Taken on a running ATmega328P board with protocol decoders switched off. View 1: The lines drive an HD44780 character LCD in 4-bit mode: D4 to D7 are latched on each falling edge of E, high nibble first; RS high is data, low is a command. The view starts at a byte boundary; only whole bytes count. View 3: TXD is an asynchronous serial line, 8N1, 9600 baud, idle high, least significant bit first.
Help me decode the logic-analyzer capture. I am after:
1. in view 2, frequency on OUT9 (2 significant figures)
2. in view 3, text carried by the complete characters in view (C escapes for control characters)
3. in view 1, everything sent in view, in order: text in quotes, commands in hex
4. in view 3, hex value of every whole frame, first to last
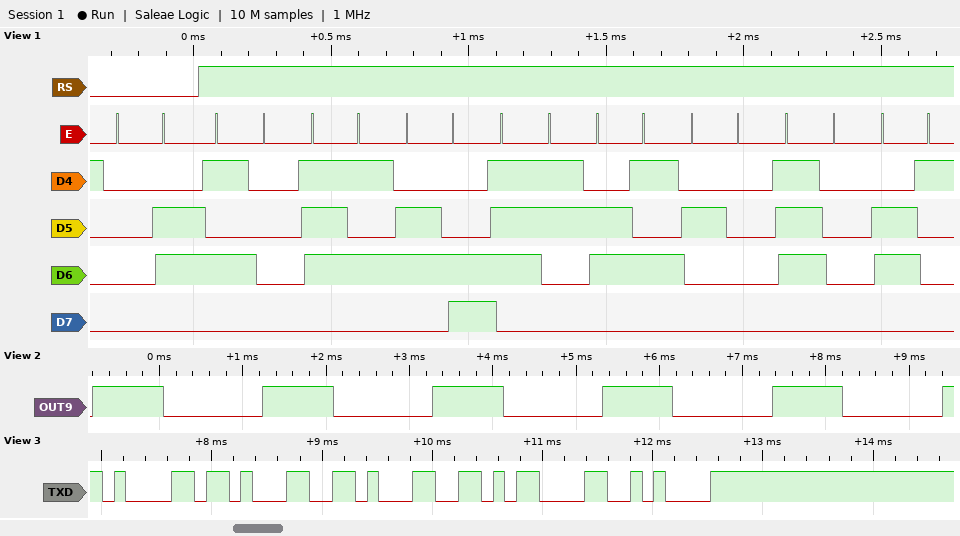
490 Hz
"a11\r\n"
0x06 "Pulse pa"
61 31 31 0D 0A
